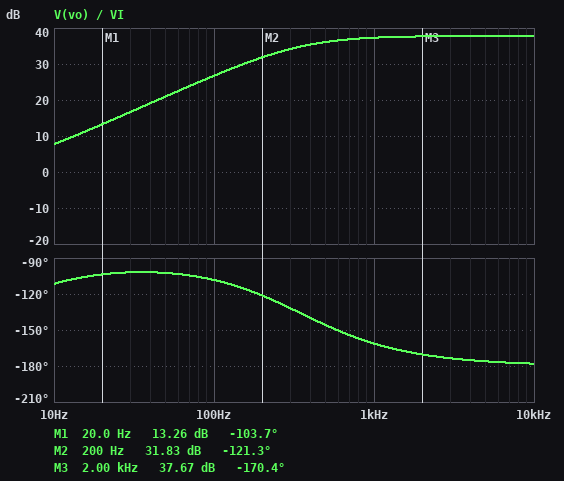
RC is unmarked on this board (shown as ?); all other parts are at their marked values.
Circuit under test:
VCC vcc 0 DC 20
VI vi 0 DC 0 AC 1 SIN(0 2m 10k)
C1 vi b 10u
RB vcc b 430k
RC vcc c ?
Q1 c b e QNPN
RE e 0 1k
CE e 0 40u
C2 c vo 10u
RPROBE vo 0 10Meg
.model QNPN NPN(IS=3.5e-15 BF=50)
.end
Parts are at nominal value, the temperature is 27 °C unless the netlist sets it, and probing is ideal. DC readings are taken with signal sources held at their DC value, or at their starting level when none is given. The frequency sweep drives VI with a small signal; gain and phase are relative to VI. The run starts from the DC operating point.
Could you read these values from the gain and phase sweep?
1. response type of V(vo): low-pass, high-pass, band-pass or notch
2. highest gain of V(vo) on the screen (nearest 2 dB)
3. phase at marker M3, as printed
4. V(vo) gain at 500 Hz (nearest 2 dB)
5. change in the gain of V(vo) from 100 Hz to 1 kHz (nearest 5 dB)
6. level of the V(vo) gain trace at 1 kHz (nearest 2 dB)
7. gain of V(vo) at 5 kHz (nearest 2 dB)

high-pass
38 dB
-170.4 deg
36 dB
10 dB
38 dB
38 dB
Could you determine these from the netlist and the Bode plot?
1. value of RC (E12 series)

1 kΩ
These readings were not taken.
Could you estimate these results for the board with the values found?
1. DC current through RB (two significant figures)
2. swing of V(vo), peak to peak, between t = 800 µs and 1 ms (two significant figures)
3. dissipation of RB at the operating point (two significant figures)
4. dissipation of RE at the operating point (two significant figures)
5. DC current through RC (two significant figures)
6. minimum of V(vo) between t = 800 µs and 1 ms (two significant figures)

40 µA
310 mV
690 µW
4.2 mW
2.0 mA
-160 mV
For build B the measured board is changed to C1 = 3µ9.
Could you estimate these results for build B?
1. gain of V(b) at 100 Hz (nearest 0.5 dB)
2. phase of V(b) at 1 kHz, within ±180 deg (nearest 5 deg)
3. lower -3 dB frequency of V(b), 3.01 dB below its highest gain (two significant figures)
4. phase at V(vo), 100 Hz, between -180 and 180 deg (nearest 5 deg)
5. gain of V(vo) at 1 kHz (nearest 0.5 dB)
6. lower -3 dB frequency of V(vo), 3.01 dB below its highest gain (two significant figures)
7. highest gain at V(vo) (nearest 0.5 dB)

-1.5 dB
5 deg
1.2 Hz
-105 deg
37.0 dB
380 Hz
38.0 dB
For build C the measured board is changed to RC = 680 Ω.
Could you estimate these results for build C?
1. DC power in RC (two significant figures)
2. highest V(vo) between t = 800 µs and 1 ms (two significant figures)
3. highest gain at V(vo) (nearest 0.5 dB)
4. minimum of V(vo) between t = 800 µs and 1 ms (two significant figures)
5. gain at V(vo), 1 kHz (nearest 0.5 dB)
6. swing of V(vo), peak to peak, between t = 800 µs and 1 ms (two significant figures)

2.7 mW
100 mV
34.5 dB
-110 mV
34.0 dB
210 mV
